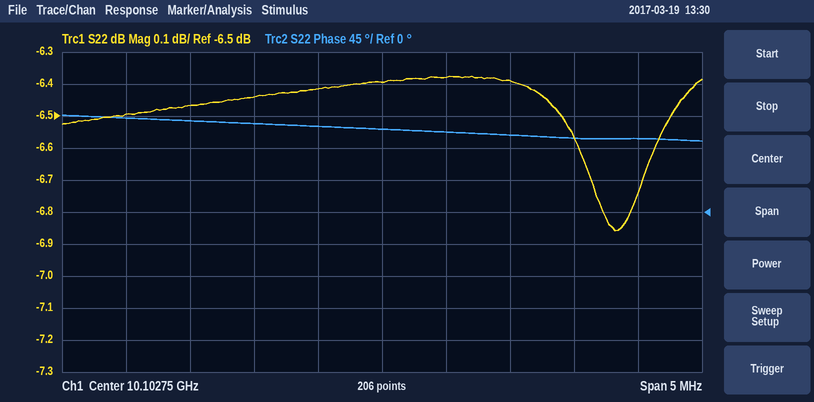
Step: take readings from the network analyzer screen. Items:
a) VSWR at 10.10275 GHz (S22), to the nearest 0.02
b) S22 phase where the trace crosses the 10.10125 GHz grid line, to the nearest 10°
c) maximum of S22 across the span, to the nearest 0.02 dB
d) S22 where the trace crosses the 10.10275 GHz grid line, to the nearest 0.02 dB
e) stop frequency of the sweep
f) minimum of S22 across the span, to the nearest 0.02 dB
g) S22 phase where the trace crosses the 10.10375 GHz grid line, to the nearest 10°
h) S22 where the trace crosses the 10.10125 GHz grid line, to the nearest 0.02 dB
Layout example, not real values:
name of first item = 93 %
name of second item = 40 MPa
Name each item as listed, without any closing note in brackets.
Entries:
VSWR at 10.10275 GHz (S22), to the nearest 0.02 = 2.84
S22 phase where the trace crosses the 10.10125 GHz grid line, to the nearest 10° = 130°
maximum of S22 across the span, to the nearest 0.02 dB = -6.38 dB
S22 where the trace crosses the 10.10275 GHz grid line, to the nearest 0.02 dB = -6.40 dB
stop frequency of the sweep = 10.10525 GHz
minimum of S22 across the span, to the nearest 0.02 dB = -6.86 dB
S22 phase where the trace crosses the 10.10375 GHz grid line, to the nearest 10° = 110°
S22 where the trace crosses the 10.10125 GHz grid line, to the nearest 0.02 dB = -6.46 dB
